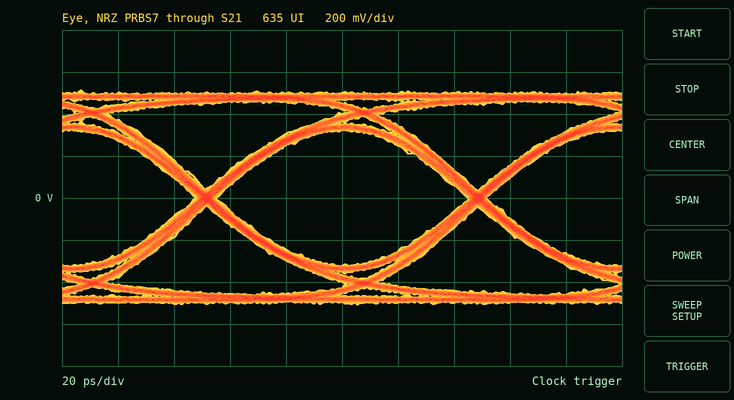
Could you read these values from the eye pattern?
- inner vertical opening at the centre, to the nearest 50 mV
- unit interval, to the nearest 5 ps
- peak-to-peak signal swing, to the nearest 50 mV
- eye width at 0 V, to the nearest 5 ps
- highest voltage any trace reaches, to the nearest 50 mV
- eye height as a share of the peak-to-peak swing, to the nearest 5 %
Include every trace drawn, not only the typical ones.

650 mV
95 ps
1.00 V
90 ps
500 mV
65 %
